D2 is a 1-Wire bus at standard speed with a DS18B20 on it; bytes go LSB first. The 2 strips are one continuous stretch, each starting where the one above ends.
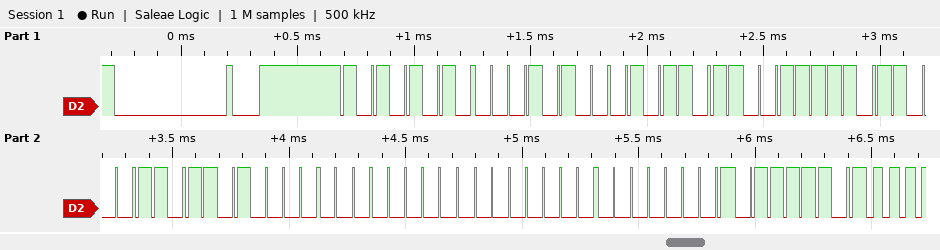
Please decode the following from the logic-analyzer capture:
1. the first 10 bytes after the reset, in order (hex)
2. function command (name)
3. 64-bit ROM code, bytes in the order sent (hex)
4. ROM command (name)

55 28 DA 7C 63 0B 00 00 80 BE
Read Scratchpad
28 DA 7C 63 0B 00 00 80
Match ROM
